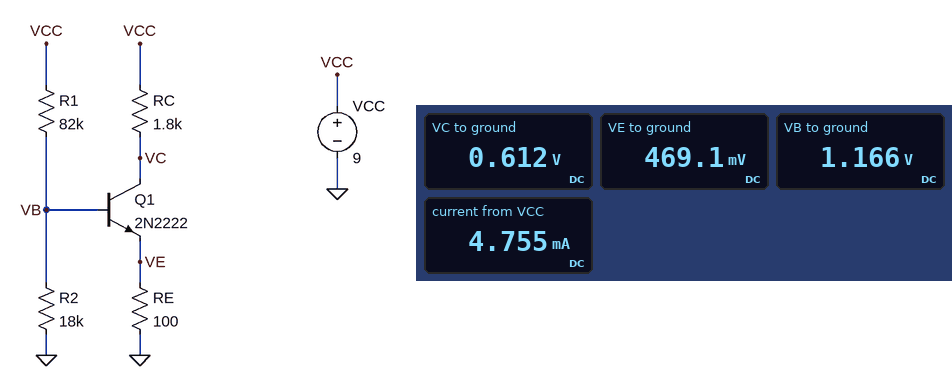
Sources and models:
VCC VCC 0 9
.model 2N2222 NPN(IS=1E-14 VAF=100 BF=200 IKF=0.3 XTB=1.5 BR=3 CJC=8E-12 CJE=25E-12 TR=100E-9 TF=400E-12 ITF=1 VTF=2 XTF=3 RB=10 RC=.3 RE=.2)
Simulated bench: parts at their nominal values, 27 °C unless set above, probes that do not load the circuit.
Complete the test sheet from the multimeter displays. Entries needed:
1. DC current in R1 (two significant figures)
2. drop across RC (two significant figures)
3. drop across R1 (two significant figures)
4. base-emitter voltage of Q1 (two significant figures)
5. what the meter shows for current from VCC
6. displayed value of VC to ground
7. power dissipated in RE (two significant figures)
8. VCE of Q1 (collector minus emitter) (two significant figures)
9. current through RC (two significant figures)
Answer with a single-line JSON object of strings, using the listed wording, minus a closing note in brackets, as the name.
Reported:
{"DC current in R1": "96 µA", "drop across RC": "8.4 V", "drop across R1": "7.8 V", "base-emitter voltage of Q1": "700 mV", "what the meter shows for current from VCC": "4.755 mA", "displayed value of VC to ground": "0.612 V", "power dissipated in RE": "2.2 mW", "VCE of Q1 (collector minus emitter)": "140 mV", "current through RC": "4.7 mA"}
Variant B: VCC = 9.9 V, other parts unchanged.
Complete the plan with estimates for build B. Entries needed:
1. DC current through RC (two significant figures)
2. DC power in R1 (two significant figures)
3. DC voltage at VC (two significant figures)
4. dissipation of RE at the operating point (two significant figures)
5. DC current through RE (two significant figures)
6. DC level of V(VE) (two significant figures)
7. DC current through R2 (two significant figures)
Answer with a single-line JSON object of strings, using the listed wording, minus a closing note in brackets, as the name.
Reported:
{"DC current through RC": "5.1 mA", "DC power in R1": "920 µW", "DC voltage at VC": "650 mV", "dissipation of RE at the operating point": "2.7 mW", "DC current through RE": "5.2 mA", "DC level of V(VE)": "520 mV", "DC current through R2": "68 µA"}
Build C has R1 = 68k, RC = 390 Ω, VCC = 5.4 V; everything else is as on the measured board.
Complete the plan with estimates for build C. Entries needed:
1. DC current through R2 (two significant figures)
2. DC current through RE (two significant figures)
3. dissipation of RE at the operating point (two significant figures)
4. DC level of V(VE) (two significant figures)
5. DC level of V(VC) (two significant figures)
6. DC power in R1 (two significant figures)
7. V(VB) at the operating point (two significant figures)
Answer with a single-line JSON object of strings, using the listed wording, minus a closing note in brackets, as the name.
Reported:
{"DC current through R2": "53 µA", "DC current through RE": "2.7 mA", "dissipation of RE at the operating point": "710 µW", "DC level of V(VE)": "270 mV", "DC level of V(VC)": "4.4 V", "DC power in R1": "290 µW", "V(VB) at the operating point": "950 mV"}
